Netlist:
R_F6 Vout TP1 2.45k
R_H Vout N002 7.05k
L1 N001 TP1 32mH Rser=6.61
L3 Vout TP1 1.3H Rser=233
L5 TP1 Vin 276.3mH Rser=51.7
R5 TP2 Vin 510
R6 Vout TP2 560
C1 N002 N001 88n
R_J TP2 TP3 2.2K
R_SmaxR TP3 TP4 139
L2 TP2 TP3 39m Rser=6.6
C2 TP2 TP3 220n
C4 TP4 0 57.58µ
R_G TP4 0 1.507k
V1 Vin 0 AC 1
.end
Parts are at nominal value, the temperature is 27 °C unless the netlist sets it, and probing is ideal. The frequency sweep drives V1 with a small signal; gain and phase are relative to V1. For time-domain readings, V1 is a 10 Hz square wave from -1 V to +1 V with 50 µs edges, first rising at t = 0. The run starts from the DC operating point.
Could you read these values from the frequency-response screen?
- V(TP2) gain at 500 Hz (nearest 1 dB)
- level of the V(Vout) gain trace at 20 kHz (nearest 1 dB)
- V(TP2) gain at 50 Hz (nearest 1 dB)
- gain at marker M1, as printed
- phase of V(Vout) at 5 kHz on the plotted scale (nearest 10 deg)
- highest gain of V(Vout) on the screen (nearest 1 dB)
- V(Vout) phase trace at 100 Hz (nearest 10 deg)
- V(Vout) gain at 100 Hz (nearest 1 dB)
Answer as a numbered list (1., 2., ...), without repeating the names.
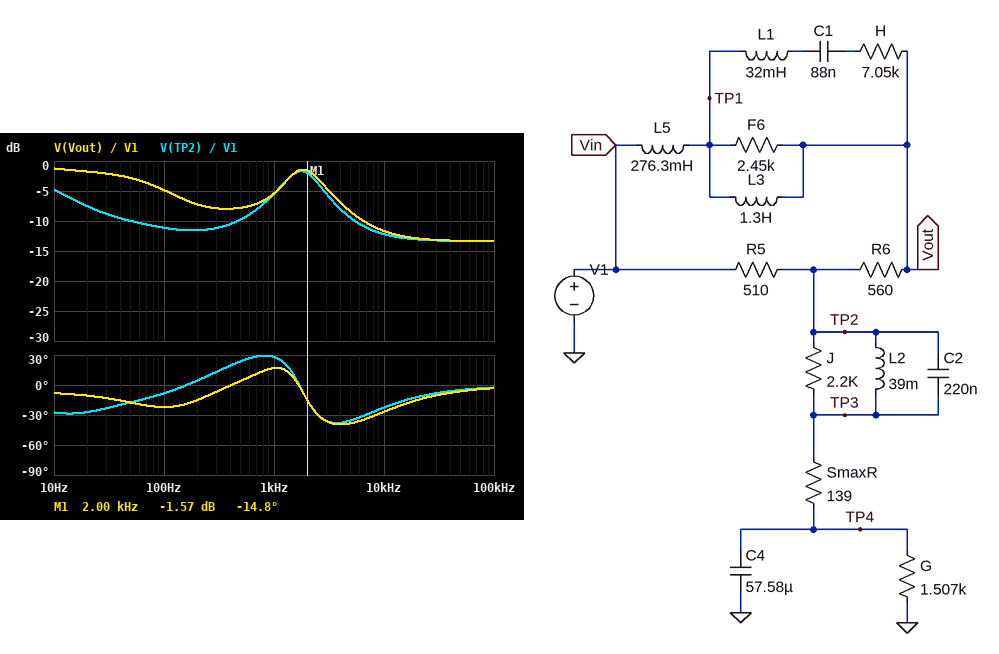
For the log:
1. -10 dB
2. -13 dB
3. -10 dB
4. -1.57 dB
5. -40 deg
6. -1 dB
7. -20 deg
8. -5 dB
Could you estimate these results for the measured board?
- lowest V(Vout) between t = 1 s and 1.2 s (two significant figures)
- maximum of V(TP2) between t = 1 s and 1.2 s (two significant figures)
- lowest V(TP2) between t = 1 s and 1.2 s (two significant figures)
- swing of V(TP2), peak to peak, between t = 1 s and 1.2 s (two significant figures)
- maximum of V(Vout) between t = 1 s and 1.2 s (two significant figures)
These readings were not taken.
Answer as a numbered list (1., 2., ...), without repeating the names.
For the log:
1. -930 mV
2. 760 mV
3. -760 mV
4. 1.5 V
5. 930 mV
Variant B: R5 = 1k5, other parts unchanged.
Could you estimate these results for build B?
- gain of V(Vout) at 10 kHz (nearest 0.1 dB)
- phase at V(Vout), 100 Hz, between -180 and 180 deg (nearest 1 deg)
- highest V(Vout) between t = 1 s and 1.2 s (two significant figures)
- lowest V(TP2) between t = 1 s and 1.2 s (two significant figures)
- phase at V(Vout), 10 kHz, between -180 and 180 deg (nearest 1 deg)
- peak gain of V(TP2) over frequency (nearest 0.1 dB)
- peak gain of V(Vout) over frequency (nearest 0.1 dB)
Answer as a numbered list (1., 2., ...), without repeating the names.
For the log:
1. -18.4 dB
2. -29 deg
3. 880 mV
4. -610 mV
5. -40 deg
6. -2.4 dB
7. -0.7 dB
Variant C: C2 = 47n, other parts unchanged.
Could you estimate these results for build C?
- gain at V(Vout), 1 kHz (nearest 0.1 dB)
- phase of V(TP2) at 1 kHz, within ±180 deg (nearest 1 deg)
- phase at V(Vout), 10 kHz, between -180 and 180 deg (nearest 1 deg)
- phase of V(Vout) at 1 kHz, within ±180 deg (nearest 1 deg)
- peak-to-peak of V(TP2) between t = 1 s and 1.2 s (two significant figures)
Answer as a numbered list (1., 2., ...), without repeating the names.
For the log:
1. -6.7 dB
2. 30 deg
3. -35 deg
4. 15 deg
5. 1.5 V
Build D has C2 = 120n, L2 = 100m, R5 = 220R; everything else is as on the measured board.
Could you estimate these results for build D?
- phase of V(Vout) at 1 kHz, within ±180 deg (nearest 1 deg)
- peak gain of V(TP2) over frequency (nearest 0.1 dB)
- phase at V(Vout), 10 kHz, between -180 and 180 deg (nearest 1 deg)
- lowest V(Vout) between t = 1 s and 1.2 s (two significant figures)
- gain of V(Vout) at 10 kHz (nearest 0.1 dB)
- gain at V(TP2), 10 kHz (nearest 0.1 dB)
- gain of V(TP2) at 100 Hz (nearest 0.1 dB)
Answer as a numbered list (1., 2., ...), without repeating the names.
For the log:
1. 6 deg
2. -0.8 dB
3. -24 deg
4. -960 mV
5. -5.6 dB
6. -5.8 dB
7. -7.1 dB
